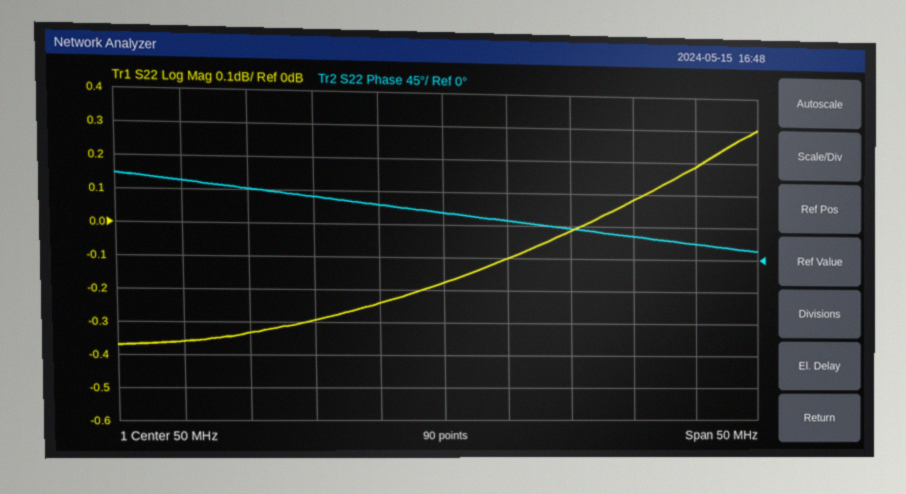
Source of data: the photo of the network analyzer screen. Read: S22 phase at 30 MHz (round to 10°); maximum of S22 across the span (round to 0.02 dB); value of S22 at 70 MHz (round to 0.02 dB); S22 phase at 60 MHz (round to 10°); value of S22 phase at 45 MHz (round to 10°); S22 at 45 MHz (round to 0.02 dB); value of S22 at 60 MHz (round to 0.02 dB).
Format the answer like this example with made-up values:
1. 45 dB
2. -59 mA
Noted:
1. 100°
2. 0.30 dB
3. 0.18 dB
4. 40°
5. 70°
6. -0.24 dB
7. -0.02 dB
